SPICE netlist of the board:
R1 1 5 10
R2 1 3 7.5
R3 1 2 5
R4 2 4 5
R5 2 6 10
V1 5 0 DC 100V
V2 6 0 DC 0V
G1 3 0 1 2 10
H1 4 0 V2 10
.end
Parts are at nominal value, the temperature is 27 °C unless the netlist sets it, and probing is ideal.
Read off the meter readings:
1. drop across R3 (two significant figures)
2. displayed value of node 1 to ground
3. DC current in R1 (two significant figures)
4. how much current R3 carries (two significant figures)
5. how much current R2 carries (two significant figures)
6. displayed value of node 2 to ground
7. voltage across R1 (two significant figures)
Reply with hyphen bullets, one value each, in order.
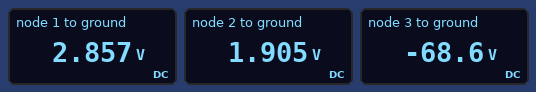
- 950 mV
- 2.857 V
- 9.7 A
- 190 mA
- 9.5 A
- 1.905 V
- 97 V
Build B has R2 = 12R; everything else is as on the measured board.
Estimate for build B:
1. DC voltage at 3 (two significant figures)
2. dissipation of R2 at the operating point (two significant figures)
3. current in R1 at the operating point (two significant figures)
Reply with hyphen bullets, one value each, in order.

- -110 V
- 1.1 kW
- 9.7 A
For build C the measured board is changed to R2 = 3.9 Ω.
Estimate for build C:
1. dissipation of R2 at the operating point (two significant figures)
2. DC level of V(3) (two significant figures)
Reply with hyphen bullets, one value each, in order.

- 350 W
- -34 V
